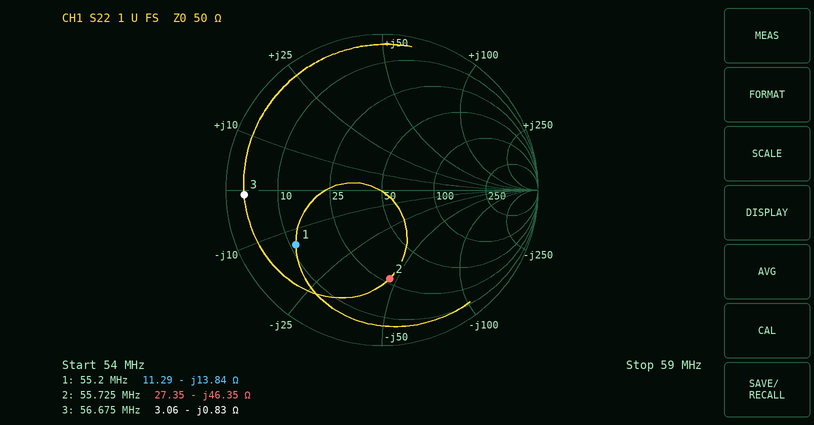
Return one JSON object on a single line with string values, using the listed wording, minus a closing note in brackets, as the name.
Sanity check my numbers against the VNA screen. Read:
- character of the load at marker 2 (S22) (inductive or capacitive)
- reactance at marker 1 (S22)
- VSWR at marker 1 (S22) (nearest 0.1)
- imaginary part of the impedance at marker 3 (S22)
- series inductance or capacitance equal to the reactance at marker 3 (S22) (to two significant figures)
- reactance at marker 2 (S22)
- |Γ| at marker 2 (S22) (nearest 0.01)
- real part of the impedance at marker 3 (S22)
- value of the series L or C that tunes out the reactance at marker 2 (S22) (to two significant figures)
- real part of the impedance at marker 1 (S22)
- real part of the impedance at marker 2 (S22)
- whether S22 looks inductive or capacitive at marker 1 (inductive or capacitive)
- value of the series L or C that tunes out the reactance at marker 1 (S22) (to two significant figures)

{"character of the load at marker 2 (S22)": "capacitive", "reactance at marker 1": "-13.84 Ω", "VSWR at marker 1 (S22)": "4.8", "imaginary part of the impedance at marker 3": "-0.83 Ω", "series inductance or capacitance equal to the reactance at marker 3 (S22)": "3.4 nF", "reactance at marker 2": "-46.35 Ω", "|Γ| at marker 2 (S22)": "0.57", "real part of the impedance at marker 3": "3.06 Ω", "value of the series L or C that tunes out the reactance at marker 2 (S22)": "130 nH", "real part of the impedance at marker 1": "11.29 Ω", "real part of the impedance at marker 2": "27.35 Ω", "whether S22 looks inductive or capacitive at marker 1": "capacitive", "value of the series L or C that tunes out the reactance at marker 1 (S22)": "40 nH"}
